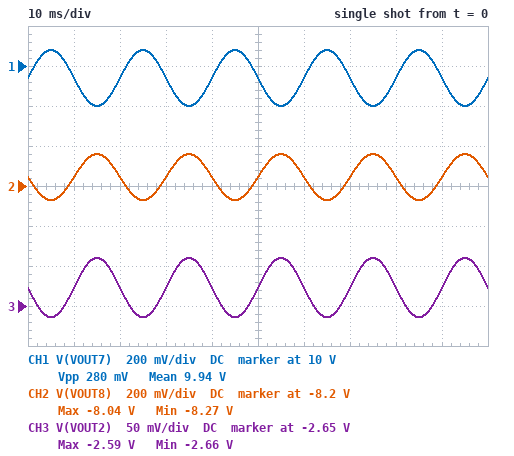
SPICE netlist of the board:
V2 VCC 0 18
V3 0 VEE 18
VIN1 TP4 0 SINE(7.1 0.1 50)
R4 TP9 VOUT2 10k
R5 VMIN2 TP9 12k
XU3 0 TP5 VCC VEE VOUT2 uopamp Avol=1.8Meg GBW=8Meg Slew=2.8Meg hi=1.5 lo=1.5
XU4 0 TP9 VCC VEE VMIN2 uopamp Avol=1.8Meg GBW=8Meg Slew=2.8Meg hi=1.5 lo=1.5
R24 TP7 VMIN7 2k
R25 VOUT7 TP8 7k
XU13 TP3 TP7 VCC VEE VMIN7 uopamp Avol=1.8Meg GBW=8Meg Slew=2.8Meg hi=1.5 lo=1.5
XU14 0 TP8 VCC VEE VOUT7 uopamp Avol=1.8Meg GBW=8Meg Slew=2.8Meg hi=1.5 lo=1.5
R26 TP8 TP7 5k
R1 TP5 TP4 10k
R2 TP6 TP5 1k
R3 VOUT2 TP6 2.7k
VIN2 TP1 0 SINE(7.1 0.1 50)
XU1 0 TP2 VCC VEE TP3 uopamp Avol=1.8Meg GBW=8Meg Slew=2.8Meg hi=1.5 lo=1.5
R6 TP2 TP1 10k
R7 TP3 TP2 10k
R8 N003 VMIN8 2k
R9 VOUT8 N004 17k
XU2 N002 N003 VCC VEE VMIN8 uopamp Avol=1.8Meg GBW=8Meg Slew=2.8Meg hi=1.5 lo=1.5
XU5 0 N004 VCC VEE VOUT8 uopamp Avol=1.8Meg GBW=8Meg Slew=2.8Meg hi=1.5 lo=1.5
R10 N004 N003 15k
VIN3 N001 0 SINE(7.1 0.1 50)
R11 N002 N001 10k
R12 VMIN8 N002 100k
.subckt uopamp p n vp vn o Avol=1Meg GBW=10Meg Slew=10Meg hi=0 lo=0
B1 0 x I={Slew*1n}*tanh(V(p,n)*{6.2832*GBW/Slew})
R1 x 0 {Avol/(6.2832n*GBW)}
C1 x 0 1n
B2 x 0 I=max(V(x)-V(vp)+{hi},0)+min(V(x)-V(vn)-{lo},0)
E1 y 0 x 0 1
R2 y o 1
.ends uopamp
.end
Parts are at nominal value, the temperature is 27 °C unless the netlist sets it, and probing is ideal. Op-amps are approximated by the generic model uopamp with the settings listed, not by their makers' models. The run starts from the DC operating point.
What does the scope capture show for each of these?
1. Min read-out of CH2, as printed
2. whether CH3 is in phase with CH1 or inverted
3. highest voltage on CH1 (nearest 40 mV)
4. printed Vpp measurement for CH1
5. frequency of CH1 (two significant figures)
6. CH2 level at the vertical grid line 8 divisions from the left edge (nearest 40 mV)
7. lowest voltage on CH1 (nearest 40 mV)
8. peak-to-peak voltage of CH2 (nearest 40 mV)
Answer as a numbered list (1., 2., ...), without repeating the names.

1. -8.27 V
2. inverted
3. 10.08 V
4. 280 mV
5. 50 Hz
6. -8.16 V
7. 9.80 V
8. 240 mV
